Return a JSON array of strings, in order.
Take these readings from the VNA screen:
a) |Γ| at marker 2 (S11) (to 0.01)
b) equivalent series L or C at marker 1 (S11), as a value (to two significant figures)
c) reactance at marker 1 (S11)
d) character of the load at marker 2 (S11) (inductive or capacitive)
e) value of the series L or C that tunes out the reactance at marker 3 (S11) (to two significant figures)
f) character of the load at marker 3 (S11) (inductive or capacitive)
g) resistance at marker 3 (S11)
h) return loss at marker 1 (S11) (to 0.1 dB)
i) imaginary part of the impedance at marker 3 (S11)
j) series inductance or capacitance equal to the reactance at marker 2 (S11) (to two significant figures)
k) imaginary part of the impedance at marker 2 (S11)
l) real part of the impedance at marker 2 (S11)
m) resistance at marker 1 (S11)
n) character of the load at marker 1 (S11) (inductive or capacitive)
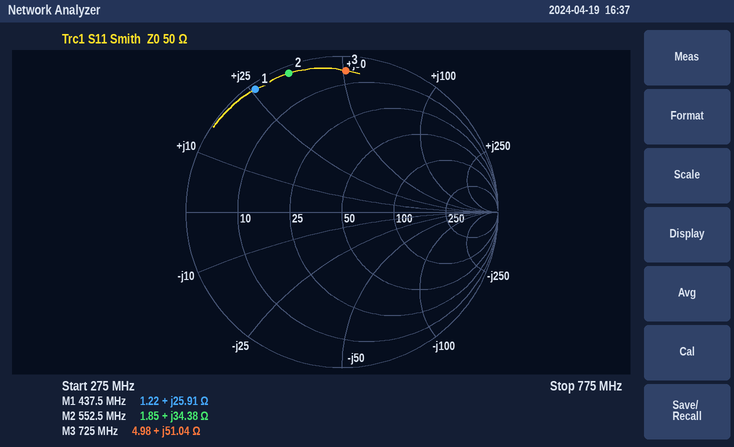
["0.95", "9.4 nH", "+25.91 Ω", "inductive", "4.3 pF", "inductive", "4.98 Ω", "0.3 dB", "+51.04 Ω", "9.9 nH", "+34.38 Ω", "1.85 Ω", "1.22 Ω", "inductive"]
